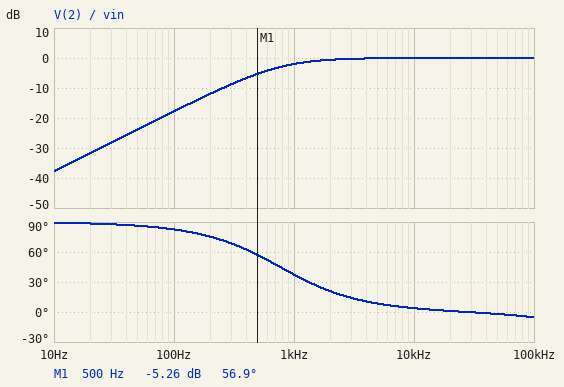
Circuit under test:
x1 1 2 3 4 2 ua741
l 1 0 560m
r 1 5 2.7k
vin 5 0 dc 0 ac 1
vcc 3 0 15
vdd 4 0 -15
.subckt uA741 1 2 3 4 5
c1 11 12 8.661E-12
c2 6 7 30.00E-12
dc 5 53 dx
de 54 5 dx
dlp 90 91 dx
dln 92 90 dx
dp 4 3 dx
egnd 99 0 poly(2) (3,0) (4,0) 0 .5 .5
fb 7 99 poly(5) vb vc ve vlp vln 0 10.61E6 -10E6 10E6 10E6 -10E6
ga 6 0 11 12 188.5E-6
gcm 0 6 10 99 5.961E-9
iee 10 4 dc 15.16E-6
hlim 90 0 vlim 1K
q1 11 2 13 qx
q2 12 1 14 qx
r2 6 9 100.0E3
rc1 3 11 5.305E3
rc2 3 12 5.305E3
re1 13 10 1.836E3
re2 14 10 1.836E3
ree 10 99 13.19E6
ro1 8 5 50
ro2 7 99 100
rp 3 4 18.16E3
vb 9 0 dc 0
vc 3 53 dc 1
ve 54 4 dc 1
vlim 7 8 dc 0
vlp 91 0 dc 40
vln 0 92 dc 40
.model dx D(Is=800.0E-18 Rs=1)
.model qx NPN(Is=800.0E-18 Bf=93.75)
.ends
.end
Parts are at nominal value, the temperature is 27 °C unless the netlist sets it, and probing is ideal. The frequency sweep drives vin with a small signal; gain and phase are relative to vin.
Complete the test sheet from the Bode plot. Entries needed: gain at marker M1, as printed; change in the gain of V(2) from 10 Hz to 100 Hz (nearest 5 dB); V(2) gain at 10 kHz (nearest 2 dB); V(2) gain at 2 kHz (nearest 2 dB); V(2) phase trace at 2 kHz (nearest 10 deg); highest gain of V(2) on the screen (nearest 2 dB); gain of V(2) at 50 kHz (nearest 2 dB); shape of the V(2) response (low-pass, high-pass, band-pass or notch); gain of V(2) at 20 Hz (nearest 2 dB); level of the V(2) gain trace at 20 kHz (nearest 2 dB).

-5.26 dB
20 dB
0 dB
0 dB
20 deg
0 dB
0 dB
high-pass
-32 dB
0 dB
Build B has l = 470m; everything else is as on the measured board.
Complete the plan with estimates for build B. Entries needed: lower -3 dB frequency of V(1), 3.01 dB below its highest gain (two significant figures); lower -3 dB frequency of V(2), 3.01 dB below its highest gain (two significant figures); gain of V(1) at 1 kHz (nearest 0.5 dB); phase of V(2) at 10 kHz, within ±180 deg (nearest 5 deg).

910 Hz
930 Hz
-2.5 dB
5 deg
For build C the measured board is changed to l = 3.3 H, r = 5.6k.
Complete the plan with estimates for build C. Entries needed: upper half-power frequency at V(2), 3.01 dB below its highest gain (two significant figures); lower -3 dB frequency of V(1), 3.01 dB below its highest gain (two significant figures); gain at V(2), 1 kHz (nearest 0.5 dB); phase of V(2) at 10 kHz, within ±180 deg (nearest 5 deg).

1.4 MHz
270 Hz
-0.5 dB
0 deg
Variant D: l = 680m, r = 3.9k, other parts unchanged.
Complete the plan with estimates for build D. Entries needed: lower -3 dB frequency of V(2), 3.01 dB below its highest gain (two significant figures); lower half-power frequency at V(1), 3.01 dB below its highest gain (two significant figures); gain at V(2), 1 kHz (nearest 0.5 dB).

930 Hz
910 Hz
-2.5 dB
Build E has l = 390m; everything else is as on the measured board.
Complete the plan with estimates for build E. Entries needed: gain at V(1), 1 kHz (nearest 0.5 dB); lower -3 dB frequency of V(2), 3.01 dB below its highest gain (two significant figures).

-3.5 dB
1.1 kHz
